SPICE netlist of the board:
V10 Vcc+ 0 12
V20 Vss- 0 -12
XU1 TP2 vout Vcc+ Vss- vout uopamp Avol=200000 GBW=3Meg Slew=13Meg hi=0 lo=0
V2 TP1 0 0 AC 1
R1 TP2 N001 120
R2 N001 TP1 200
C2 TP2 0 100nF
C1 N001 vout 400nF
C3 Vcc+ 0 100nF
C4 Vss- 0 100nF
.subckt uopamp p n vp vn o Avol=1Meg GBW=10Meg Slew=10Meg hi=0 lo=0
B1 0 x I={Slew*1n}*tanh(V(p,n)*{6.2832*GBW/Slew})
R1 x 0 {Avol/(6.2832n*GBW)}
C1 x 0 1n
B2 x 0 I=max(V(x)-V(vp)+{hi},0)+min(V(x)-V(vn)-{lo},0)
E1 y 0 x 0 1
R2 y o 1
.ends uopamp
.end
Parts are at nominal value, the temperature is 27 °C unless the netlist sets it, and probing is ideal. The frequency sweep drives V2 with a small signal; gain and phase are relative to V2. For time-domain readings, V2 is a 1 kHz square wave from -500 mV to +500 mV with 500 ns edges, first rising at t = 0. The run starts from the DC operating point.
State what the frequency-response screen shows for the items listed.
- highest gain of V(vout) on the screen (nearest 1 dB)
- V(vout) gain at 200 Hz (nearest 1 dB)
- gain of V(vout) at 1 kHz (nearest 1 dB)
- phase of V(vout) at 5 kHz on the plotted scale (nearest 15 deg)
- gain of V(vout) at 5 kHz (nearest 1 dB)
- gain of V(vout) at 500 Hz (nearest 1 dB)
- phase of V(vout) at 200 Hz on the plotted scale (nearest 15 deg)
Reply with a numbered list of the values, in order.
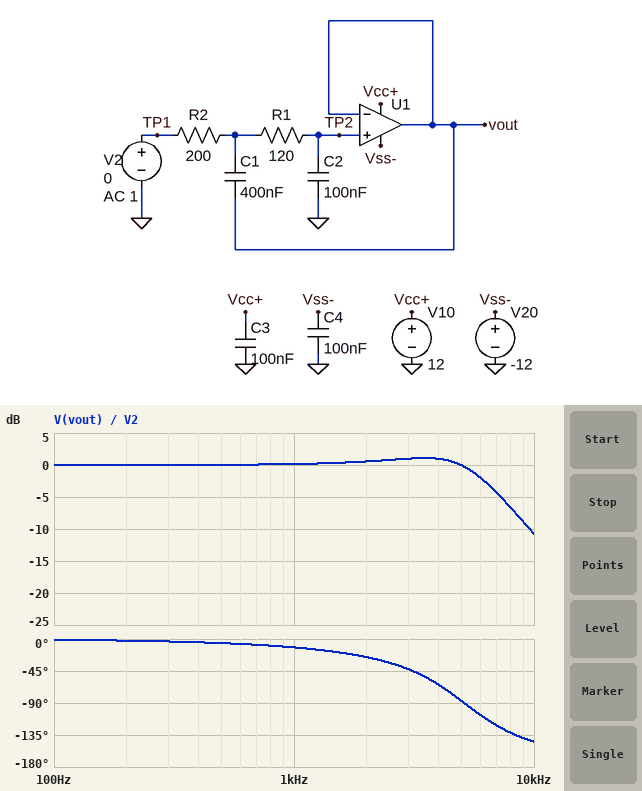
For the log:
1. 1 dB
2. 0 dB
3. 0 dB
4. -90 deg
5. 0 dB
6. 0 dB
7. 0 deg
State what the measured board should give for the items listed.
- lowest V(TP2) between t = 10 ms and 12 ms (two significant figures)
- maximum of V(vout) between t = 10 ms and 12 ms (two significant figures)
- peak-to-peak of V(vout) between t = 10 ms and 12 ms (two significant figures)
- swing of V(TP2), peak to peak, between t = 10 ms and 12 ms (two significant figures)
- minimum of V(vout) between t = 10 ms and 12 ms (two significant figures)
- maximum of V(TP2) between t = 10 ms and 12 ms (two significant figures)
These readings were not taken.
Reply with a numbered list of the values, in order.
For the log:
1. -650 mV
2. 650 mV
3. 1.3 V
4. 1.3 V
5. -650 mV
6. 650 mV
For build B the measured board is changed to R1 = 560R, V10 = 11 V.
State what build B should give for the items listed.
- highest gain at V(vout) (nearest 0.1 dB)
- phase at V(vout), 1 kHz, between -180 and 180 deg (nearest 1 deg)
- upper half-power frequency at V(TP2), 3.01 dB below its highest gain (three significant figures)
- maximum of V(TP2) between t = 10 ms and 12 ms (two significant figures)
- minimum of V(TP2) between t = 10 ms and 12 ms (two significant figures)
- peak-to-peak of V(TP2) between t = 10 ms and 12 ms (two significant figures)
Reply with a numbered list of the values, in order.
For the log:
1. 0.6 dB
2. -30 deg
3. 2.70 kHz
4. 610 mV
5. -610 mV
6. 1.2 V
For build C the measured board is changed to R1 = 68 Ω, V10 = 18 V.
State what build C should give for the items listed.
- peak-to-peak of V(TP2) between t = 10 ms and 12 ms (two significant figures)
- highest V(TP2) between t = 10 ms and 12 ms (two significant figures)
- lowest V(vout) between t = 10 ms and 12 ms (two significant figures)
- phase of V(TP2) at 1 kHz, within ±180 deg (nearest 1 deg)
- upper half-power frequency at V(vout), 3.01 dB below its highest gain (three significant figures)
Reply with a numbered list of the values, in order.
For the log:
1. 1.2 V
2. 610 mV
3. -610 mV
4. -10 deg
5. 7.70 kHz
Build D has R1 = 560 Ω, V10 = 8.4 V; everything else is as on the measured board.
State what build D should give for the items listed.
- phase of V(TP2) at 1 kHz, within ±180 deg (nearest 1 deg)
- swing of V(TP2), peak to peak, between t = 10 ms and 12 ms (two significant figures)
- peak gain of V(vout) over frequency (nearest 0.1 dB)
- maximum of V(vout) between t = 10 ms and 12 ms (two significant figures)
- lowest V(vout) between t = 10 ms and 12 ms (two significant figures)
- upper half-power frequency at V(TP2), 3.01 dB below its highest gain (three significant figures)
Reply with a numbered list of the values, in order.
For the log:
1. -30 deg
2. 1.2 V
3. 0.6 dB
4. 610 mV
5. -610 mV
6. 2.70 kHz
